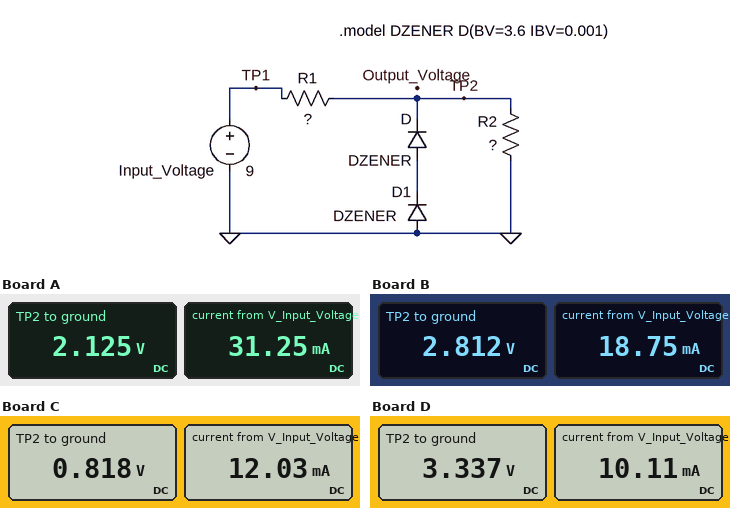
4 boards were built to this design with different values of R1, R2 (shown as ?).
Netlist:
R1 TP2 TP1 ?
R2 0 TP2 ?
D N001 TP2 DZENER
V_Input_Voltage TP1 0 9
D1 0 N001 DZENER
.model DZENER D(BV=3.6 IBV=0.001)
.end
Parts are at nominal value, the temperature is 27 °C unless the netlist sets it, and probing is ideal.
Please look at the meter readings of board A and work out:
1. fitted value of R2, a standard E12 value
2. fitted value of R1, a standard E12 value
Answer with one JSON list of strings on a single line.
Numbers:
["68 Ω", "220 Ω"]
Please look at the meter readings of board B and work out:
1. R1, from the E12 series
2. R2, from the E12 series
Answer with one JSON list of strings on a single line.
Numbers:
["330 Ω", "150 Ω"]
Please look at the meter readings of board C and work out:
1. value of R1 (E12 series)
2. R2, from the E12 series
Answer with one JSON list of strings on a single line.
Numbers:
["680 Ω", "68 Ω"]
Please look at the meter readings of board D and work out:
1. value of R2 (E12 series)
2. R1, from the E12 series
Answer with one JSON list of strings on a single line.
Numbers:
["330 Ω", "560 Ω"]
